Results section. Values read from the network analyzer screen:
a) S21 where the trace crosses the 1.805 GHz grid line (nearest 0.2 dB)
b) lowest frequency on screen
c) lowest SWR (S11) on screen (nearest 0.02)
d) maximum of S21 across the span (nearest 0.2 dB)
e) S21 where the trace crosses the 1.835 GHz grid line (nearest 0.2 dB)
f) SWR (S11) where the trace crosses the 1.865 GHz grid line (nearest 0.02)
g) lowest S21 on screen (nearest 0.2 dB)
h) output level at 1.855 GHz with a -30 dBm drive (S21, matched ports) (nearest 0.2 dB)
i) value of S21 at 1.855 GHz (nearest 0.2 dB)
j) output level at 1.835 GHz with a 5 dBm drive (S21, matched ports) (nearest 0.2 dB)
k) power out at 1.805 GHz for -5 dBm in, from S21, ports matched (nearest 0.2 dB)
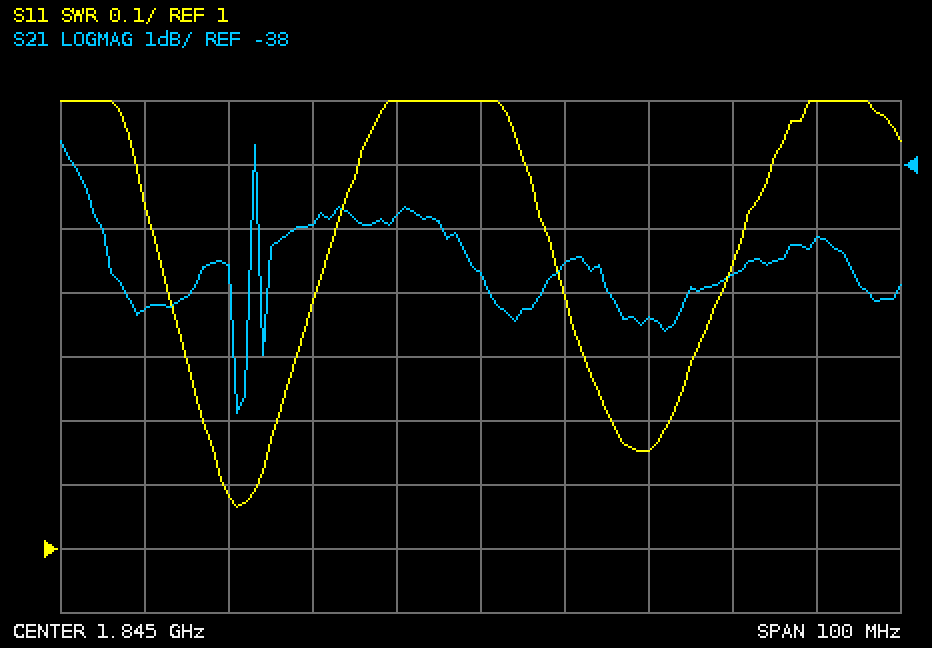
-40.2 dB
1.795 GHz
1.06
-37.6 dB
-38.8 dB
1.16
-41.8 dB
-69.6 dBm
-39.6 dB
-33.8 dBm
-45.2 dBm
